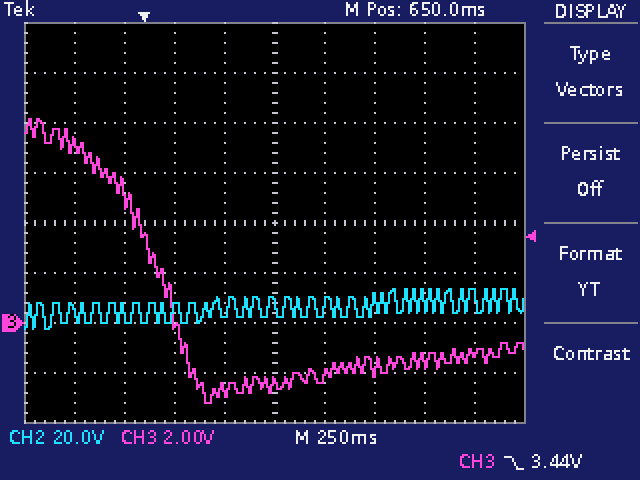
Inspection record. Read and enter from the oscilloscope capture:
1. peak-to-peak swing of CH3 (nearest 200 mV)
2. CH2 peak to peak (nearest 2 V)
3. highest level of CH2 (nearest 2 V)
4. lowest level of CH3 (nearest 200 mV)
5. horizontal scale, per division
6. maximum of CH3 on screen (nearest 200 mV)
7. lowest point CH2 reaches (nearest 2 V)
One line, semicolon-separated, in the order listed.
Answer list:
11.4 V; 16 V; 14 V; -3.2 V; 250 ms; 8.2 V; -2 V
